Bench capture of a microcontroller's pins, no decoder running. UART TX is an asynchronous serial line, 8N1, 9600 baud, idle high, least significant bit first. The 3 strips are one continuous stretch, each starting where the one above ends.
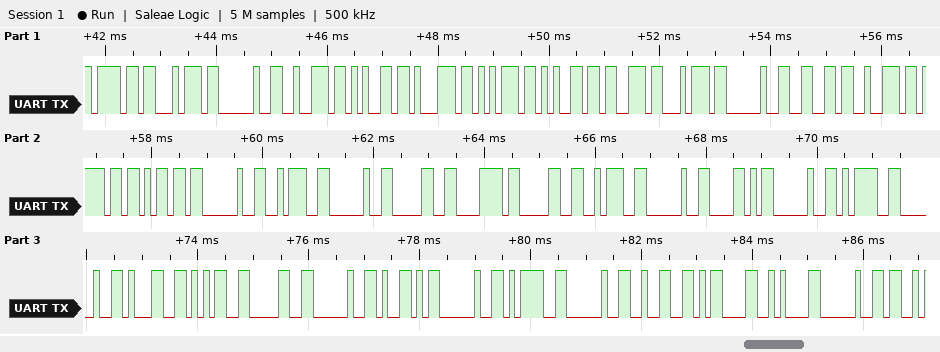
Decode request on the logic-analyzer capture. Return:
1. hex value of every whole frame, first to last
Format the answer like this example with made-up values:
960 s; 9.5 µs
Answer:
6F 74 20 72 65 71 75 65 73 74 20 66 72 6F 6D 20 3A 20 30 78 30 3A 20 58 20 3D 20 31 35 30 20 59 20 3D 20 32 0D 0A 20
